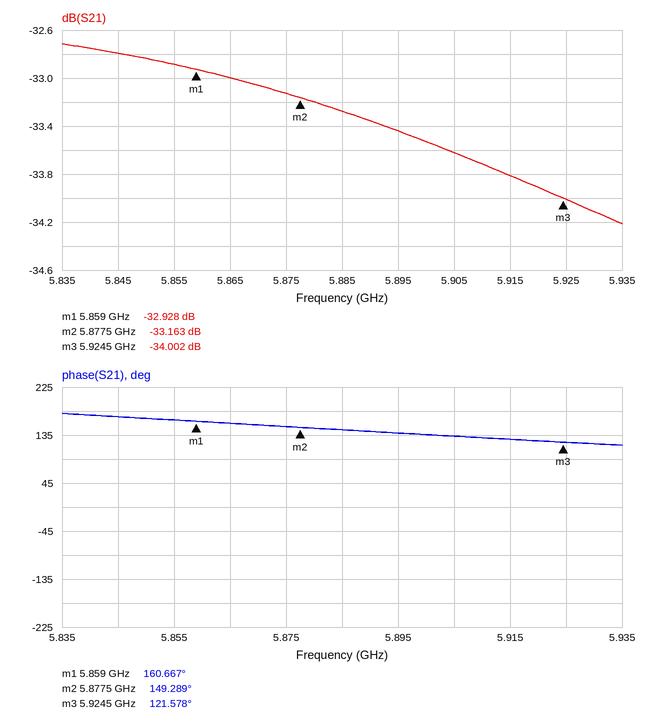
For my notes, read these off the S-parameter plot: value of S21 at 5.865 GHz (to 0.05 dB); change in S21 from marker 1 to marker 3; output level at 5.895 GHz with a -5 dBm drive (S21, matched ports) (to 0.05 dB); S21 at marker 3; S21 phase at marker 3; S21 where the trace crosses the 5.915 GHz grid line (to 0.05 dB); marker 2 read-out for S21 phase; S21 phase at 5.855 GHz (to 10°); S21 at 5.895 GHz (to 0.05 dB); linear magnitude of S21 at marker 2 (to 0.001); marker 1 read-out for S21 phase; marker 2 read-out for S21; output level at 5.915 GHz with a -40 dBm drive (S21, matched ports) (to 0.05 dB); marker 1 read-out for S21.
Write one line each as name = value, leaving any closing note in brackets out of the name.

value of S21 at 5.865 GHz = -33.00 dB
change in S21 from marker 1 to marker 3 = -1.074 dB
output level at 5.895 GHz with a -5 dBm drive (S21, matched ports) = -38.45 dBm
S21 at marker 3 = -34.002 dB
S21 phase at marker 3 = 121.578°
S21 where the trace crosses the 5.915 GHz grid line = -33.80 dB
marker 2 read-out for S21 phase = 149.289°
S21 phase at 5.855 GHz = 160°
S21 at 5.895 GHz = -33.45 dB
linear magnitude of S21 at marker 2 = 0.022
marker 1 read-out for S21 phase = 160.667°
marker 2 read-out for S21 = -33.163 dB
output level at 5.915 GHz with a -40 dBm drive (S21, matched ports) = -73.80 dBm
marker 1 read-out for S21 = -32.928 dB
